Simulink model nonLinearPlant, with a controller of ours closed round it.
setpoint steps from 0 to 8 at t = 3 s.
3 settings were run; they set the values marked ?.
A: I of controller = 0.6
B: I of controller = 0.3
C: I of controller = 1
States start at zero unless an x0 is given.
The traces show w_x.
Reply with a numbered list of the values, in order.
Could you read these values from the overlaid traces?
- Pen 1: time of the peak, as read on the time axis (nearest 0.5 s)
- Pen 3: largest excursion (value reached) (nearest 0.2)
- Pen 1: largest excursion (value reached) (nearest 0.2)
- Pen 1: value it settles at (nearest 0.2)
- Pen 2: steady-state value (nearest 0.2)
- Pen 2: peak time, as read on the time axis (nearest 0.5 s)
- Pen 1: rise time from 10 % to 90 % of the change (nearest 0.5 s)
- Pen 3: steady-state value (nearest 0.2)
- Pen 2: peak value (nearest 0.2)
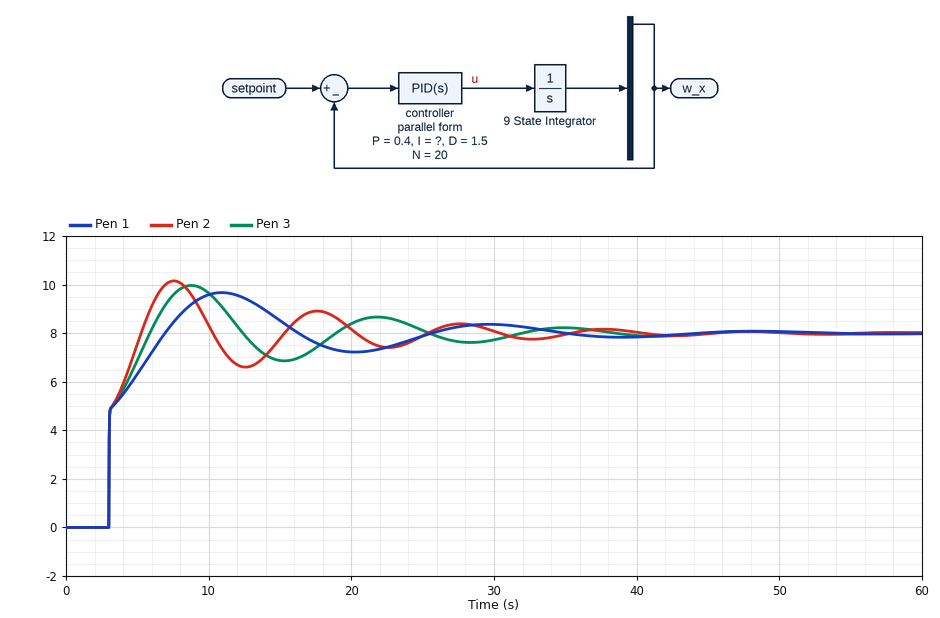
1. 11.0 s
2. 10.0
3. 9.6
4. 8.0
5. 8.0
6. 7.5 s
7. 3.0 s
8. 8.0
9. 10.2
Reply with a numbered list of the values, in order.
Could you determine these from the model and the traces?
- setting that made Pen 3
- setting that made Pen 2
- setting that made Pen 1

1. A
2. C
3. B
